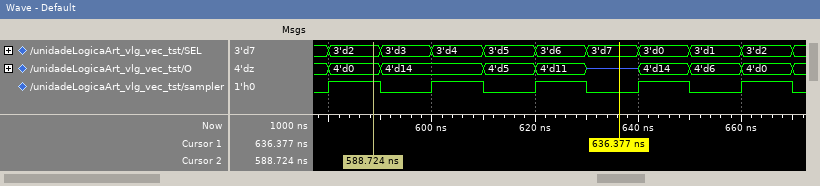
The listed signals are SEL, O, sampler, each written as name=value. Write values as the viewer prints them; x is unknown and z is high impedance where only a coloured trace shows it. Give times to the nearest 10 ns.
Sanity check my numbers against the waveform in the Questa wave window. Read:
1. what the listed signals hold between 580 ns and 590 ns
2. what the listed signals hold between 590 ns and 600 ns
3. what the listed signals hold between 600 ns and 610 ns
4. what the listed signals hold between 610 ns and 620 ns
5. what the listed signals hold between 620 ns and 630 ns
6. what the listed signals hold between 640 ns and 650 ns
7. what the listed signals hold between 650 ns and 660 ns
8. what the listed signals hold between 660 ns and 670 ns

SEL=3'd2, O=4'd0, sampler=1
SEL=3'd3, O=4'd14, sampler=0
SEL=3'd4, O=4'd14, sampler=1
SEL=3'd5, O=4'd5, sampler=0
SEL=3'd6, O=4'd11, sampler=1
SEL=3'd0, O=4'd14, sampler=1
SEL=3'd1, O=4'd6, sampler=0
SEL=3'd2, O=4'd0, sampler=1
